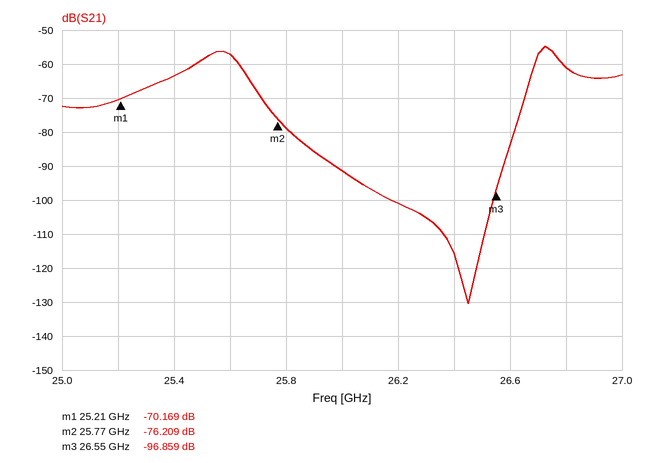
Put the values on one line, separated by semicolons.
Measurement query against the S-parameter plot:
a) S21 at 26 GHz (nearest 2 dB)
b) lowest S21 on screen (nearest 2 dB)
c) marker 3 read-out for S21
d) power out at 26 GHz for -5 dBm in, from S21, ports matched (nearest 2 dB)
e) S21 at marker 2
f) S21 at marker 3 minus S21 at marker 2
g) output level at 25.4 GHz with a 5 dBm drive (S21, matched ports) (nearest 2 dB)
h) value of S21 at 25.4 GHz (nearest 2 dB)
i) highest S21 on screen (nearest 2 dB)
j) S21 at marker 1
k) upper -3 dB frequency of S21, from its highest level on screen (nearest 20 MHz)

-92 dB; -130 dB; -96.859 dB; -96 dBm; -76.209 dB; -20.650 dB; -58 dBm; -64 dB; -54 dB; -70.169 dB; 26.76 GHz
